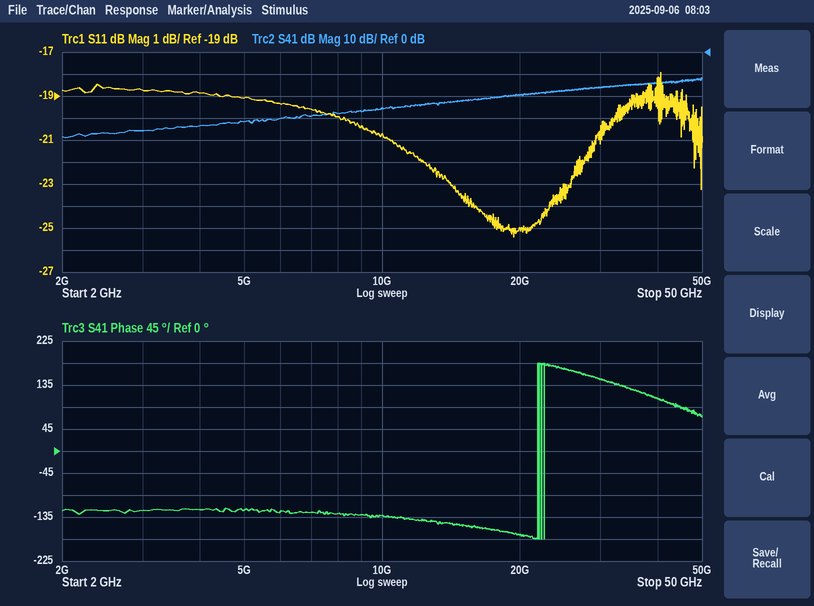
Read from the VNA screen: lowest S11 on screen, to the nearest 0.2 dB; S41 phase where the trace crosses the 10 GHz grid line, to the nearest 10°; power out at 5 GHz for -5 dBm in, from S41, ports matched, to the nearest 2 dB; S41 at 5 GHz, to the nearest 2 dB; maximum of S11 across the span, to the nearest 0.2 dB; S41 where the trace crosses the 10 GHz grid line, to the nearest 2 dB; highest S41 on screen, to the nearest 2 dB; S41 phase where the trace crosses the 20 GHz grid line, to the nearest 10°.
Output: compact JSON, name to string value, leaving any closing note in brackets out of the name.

{"lowest S11 on screen, to the nearest 0.2 dB": "-25.4 dB", "S41 phase where the trace crosses the 10 GHz grid line, to the nearest 10°": "-130°", "power out at 5 GHz for -5 dBm in, from S41, ports matched, to the nearest 2 dB": "-36 dBm", "S41 at 5 GHz, to the nearest 2 dB": "-32 dB", "maximum of S11 across the span, to the nearest 0.2 dB": "-18.0 dB", "S41 where the trace crosses the 10 GHz grid line, to the nearest 2 dB": "-26 dB", "highest S41 on screen, to the nearest 2 dB": "-12 dB", "S41 phase where the trace crosses the 20 GHz grid line, to the nearest 10°": "-170°"}
